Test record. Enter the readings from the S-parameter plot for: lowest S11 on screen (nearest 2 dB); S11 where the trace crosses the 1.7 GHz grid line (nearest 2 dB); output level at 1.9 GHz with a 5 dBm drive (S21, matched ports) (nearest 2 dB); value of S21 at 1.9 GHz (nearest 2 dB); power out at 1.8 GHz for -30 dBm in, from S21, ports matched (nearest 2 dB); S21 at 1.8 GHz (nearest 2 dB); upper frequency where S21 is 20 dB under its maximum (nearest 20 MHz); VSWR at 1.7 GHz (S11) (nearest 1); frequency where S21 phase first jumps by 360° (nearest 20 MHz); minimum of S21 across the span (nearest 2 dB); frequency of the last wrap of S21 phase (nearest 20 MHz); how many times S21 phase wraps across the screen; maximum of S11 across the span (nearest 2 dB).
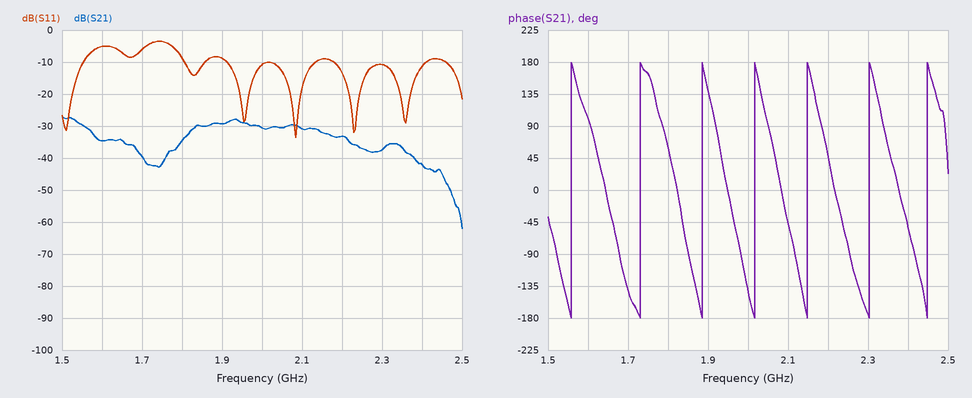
-34 dB
-6 dB
-24 dBm
-30 dB
-64 dBm
-34 dB
2.46 GHz
3
1.56 GHz
-62 dB
2.44 GHz
7
-4 dB
